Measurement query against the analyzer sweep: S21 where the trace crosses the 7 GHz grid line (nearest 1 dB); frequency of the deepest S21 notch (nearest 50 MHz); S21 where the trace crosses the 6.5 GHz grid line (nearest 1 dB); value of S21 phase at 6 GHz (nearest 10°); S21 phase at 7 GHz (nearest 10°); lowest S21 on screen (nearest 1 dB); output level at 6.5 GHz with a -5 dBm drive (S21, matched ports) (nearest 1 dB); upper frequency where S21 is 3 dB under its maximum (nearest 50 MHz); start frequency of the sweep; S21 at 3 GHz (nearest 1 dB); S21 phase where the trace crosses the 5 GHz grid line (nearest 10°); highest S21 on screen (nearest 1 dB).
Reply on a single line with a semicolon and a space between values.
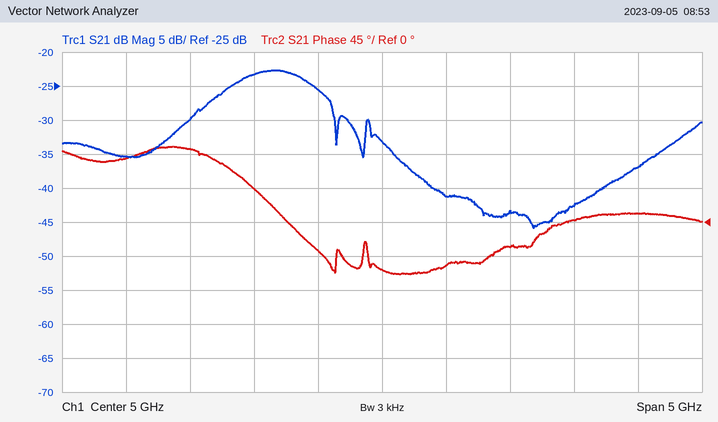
-37 dB; 6.20 GHz; -43 dB; -30°; 10°; -46 dB; -48 dBm; 4.50 GHz; 2.5 GHz; -35 dB; -60°; -23 dB
